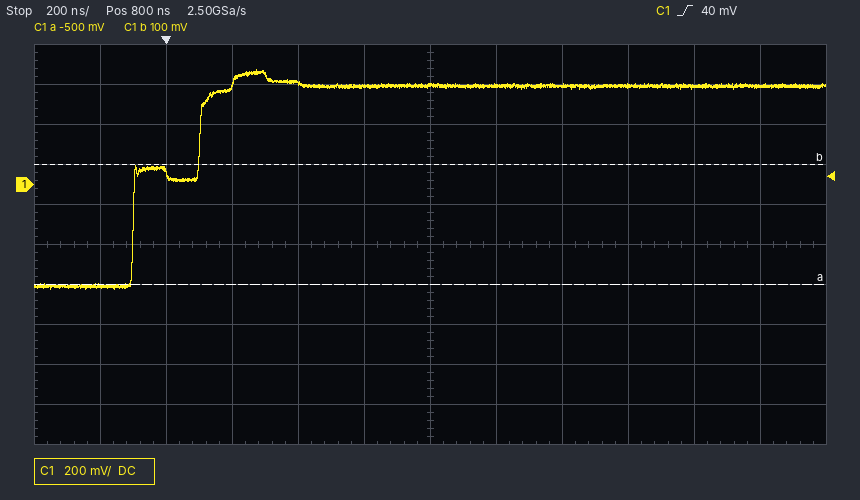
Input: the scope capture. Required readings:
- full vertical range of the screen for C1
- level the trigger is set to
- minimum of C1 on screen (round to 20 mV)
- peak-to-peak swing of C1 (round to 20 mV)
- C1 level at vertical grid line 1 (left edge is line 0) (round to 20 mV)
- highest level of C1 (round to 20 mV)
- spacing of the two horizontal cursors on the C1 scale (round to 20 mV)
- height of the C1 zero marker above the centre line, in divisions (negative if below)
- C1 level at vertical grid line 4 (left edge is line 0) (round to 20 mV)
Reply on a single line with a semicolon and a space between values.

2 V; 40 mV; -520 mV; 1.10 V; -500 mV; 580 mV; 600 mV; +1.5 div; 500 mV
